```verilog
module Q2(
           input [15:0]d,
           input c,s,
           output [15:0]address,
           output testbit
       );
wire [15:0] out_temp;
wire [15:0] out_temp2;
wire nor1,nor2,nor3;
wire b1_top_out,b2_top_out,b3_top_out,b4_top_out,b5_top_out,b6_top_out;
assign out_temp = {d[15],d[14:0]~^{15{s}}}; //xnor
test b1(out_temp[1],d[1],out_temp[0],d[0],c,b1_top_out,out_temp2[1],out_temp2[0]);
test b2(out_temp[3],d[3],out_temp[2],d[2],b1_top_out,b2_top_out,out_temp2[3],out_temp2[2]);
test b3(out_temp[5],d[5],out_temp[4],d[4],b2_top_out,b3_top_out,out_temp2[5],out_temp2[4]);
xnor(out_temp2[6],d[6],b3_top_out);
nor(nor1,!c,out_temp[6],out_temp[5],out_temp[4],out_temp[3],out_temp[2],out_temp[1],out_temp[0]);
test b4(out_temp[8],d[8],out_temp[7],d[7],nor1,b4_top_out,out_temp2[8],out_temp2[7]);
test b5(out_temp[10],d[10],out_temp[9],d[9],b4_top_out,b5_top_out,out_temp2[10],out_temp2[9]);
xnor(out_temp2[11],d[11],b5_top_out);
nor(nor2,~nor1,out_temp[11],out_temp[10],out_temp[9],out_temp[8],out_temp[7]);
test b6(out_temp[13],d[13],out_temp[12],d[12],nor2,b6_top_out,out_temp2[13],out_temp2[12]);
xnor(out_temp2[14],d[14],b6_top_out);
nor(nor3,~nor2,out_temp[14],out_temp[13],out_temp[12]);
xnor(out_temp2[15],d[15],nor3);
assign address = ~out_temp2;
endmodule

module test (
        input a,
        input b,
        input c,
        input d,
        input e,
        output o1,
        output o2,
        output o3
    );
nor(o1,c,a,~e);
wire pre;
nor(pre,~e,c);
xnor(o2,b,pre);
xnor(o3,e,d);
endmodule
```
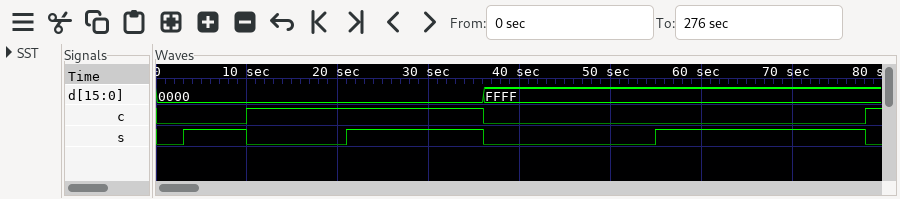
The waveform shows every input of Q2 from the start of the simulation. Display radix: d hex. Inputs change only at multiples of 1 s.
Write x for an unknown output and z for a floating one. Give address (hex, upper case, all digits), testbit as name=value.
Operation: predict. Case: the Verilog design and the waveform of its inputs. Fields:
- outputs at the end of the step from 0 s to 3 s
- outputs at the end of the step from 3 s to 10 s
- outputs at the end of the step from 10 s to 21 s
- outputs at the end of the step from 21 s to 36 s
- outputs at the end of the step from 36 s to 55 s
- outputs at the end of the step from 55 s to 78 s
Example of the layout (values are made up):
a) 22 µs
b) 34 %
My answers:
a) address=0000, testbit=z
b) address=0000, testbit=z
c) address=0001, testbit=z
d) address=FFFF, testbit=z
e) address=FFFF, testbit=z
f) address=FFFF, testbit=z
